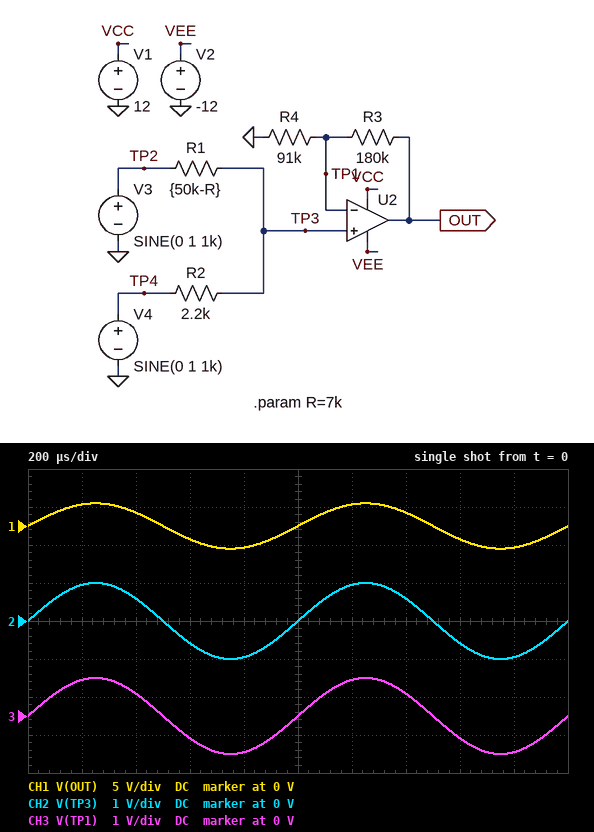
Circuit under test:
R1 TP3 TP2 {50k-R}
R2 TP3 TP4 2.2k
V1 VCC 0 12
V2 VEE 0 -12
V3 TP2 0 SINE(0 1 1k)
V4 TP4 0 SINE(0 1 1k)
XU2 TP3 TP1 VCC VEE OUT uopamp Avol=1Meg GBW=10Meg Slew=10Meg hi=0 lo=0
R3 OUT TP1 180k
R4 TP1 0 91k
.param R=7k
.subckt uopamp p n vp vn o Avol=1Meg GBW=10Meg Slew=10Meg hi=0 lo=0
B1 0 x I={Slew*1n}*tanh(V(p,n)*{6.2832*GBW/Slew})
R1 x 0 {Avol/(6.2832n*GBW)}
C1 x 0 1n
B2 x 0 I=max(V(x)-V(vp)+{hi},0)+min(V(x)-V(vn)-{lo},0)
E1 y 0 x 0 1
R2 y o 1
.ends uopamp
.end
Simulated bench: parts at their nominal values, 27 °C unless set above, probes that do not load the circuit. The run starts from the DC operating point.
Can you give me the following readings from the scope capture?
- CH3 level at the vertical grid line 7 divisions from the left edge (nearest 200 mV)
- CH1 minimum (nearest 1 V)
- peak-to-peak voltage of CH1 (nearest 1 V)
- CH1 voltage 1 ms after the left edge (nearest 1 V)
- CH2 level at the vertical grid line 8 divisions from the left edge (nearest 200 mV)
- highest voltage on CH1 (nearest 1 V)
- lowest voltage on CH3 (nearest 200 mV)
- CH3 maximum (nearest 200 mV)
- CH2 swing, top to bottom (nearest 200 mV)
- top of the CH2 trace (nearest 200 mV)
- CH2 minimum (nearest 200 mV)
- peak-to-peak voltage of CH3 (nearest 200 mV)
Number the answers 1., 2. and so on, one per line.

1. 600 mV
2. -3 V
3. 6 V
4. 0 V
5. -600 mV
6. 3 V
7. -1.0 V
8. 1.0 V
9. 2.0 V
10. 1.0 V
11. -1.0 V
12. 2.0 V
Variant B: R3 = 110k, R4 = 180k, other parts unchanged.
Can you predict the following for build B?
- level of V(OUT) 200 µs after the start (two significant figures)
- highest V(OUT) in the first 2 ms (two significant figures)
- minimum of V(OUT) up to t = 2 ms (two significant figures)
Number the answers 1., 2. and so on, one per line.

1. 1.5 V
2. 1.6 V
3. -1.6 V
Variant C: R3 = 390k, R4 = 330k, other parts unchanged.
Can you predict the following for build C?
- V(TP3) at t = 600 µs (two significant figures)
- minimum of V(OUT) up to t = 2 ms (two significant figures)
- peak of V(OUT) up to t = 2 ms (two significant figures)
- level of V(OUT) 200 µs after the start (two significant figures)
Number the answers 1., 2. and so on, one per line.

1. -590 mV
2. -2.2 V
3. 2.2 V
4. 2.1 V
